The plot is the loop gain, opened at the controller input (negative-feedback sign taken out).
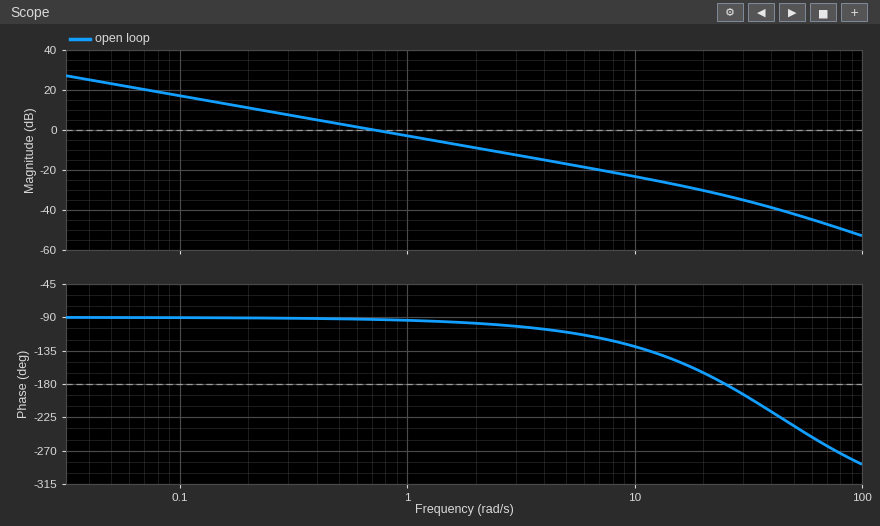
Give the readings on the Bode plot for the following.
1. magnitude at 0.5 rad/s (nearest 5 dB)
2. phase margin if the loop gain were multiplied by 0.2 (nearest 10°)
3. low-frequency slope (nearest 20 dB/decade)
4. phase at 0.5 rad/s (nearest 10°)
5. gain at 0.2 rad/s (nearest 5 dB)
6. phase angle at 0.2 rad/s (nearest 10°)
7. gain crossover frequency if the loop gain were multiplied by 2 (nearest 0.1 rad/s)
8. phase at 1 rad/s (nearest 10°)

5 dB
90°
-20 dB/decade
-90°
10 dB
-90°
1.4 rad/s
-90°
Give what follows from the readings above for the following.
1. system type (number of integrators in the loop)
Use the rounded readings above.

1
